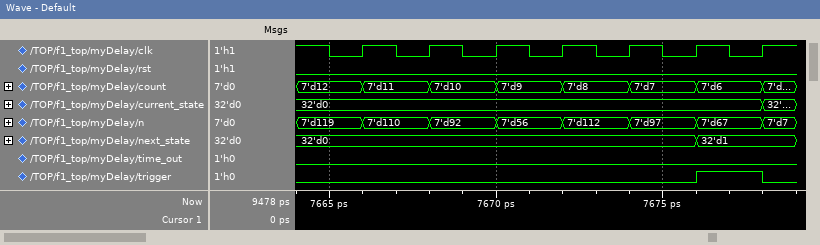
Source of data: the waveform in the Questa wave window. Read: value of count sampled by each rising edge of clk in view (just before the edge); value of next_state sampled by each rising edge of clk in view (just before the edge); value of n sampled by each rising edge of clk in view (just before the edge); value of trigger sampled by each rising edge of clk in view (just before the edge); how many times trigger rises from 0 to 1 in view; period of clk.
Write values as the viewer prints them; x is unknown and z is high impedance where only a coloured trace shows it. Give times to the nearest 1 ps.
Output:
7'd12, 7'd11, 7'd10, 7'd9, 7'd8, 7'd7, 7'd6
32'd0, 32'd0, 32'd0, 32'd0, 32'd0, 32'd0, 32'd1
7'd119, 7'd110, 7'd92, 7'd56, 7'd112, 7'd97, 7'd67
0 0 0 0 0 0 1
1
2 ps
